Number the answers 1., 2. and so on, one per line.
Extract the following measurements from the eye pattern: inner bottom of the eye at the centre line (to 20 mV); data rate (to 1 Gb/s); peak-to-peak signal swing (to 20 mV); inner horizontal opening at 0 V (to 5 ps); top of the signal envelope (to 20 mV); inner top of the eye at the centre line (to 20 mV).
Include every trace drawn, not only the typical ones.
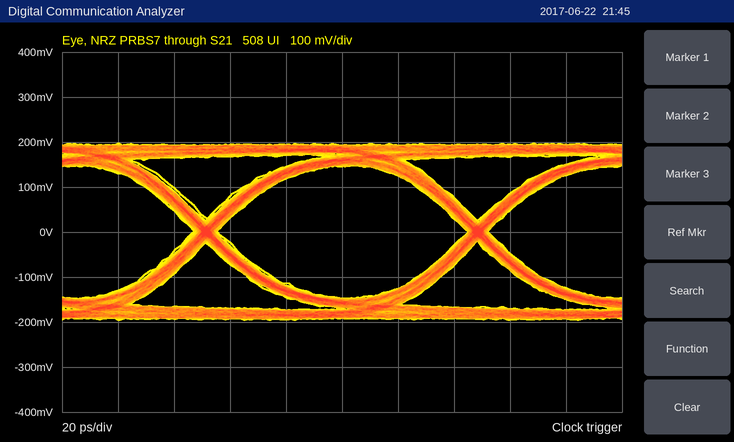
1. -140 mV
2. 10 Gb/s
3. 400 mV
4. 90 ps
5. 200 mV
6. 140 mV
